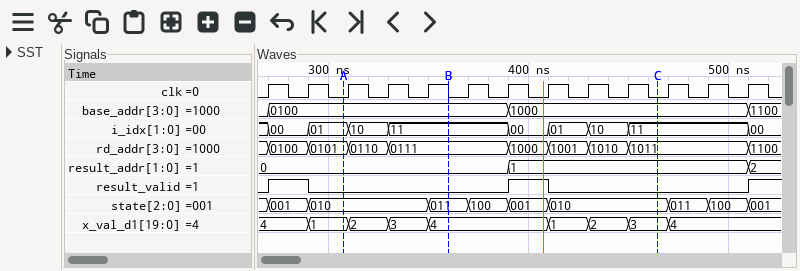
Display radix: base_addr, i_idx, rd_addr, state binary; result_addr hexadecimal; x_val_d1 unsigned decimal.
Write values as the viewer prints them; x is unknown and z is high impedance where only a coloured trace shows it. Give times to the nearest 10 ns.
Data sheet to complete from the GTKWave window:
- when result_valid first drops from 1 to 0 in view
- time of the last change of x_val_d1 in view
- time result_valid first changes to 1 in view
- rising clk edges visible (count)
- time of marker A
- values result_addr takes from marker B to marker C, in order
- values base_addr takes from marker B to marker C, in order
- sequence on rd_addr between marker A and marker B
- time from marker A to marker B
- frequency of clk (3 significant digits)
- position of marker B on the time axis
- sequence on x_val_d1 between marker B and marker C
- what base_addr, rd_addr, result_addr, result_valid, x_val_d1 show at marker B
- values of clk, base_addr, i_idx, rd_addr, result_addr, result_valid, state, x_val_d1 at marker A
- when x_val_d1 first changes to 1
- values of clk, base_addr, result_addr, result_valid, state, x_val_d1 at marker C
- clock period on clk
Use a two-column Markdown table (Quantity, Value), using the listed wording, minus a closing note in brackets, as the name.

| Quantity | Value |
|---|---|
| when result_valid first drops from 1 to 0 in view | 290 ns |
| time of the last change of x_val_d1 in view | 470 ns |
| time result_valid first changes to 1 in view | 270 ns |
| rising clk edges visible | 13 |
| time of marker A | 310 ns |
| values result_addr takes from marker B to marker C, in order | 0, 1 |
| values base_addr takes from marker B to marker C, in order | 0100, 1000 |
| sequence on rd_addr between marker A and marker B | 0101, 0110, 0111 |
| time from marker A to marker B | 50 ns |
| frequency of clk | 50.0 MHz |
| position of marker B on the time axis | 360 ns |
| sequence on x_val_d1 between marker B and marker C | 4, 1, 2, 3 |
| what base_addr, rd_addr, result_addr, result_valid, x_val_d1 show at marker B | base_addr=0100, rd_addr=0111, result_addr=0, result_valid=0, x_val_d1=4 |
| values of clk, base_addr, i_idx, rd_addr, result_addr, result_valid, state, x_val_d1 at marker A | clk=0, base_addr=0100, i_idx=01, rd_addr=0101, result_addr=0, result_valid=0, state=010, x_val_d1=1 |
| when x_val_d1 first changes to 1 | 290 ns |
| values of clk, base_addr, result_addr, result_valid, state, x_val_d1 at marker C | clk=0, base_addr=1000, result_addr=1, result_valid=0, state=010, x_val_d1=3 |
| clock period on clk | 20 ns |
